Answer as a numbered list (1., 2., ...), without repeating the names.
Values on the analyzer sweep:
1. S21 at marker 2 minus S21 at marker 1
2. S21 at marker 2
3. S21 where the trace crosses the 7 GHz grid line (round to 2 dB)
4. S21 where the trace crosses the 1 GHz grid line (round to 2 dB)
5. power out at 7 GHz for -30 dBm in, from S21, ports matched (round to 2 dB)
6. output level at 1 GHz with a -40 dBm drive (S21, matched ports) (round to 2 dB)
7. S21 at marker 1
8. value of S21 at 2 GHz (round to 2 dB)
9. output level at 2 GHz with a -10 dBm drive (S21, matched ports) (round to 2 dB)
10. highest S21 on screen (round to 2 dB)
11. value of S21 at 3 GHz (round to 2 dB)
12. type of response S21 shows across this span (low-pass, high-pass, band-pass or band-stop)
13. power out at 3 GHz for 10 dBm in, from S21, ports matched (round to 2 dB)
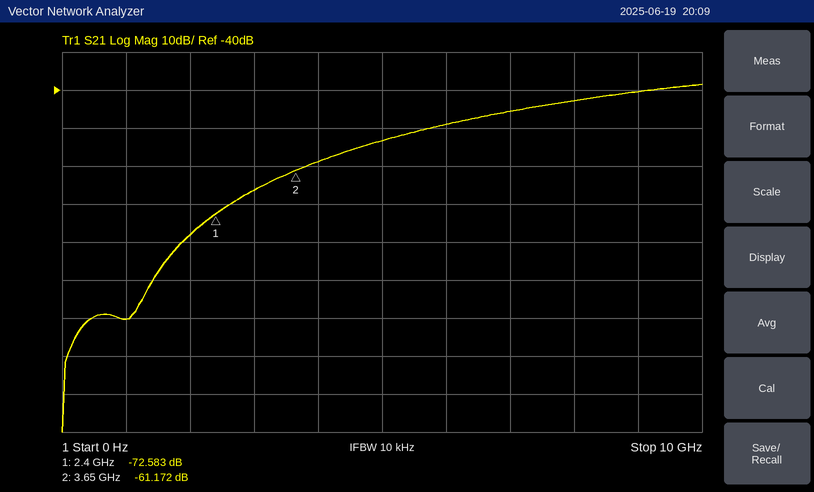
1. 11.411 dB
2. -61.172 dB
3. -46 dB
4. -100 dB
5. -76 dBm
6. -140 dBm
7. -72.583 dB
8. -78 dB
9. -88 dBm
10. -38 dB
11. -66 dB
12. high-pass
13. -56 dBm
